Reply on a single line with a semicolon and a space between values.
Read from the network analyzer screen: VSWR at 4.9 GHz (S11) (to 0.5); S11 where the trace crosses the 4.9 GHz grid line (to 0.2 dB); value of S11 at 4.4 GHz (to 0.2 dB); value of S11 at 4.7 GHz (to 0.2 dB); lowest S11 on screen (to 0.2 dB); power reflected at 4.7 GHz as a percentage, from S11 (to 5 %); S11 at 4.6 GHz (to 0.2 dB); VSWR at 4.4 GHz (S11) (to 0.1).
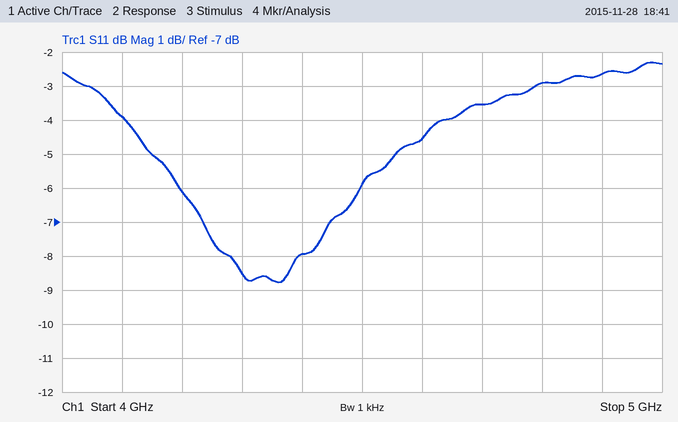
6.5; -2.6 dB; -8.0 dB; -3.6 dB; -8.8 dB; 45 %; -4.6 dB; 2.3
